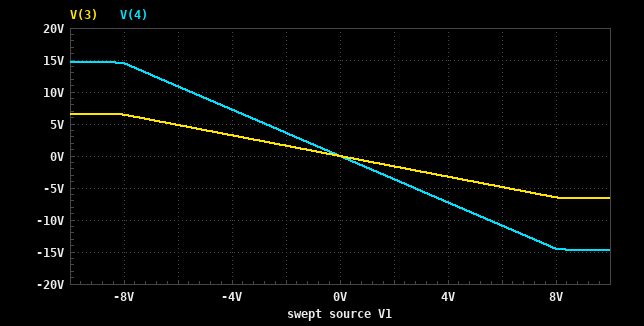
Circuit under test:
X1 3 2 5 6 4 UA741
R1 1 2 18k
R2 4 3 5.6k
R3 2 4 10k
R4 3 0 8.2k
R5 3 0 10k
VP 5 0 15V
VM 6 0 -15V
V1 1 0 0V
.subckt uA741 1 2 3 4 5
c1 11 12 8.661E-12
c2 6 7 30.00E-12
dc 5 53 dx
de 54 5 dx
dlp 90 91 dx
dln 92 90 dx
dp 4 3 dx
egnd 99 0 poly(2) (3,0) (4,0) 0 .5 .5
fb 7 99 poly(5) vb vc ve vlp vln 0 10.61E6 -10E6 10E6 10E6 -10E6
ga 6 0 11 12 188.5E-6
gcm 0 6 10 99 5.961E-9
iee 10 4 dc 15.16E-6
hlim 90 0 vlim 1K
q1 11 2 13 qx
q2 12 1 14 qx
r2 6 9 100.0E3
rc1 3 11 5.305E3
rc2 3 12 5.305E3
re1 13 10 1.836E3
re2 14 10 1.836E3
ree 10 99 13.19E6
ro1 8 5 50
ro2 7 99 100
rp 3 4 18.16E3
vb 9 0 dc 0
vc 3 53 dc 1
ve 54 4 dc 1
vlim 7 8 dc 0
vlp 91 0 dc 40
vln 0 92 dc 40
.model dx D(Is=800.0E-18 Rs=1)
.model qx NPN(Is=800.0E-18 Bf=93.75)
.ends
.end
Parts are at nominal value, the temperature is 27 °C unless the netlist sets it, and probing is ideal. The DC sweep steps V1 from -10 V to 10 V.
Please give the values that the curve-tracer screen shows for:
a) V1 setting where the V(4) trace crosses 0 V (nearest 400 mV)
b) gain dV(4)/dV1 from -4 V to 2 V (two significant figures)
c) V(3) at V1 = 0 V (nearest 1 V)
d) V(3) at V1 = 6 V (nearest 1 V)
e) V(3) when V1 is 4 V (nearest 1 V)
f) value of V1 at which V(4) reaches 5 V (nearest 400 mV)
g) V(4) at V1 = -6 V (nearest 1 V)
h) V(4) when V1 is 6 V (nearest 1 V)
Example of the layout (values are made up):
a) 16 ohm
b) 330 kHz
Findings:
a) 0 V
b) -1.8 V/V
c) 0 V
d) -5 V
e) -3 V
f) -2.8 V
g) 11 V
h) -11 V
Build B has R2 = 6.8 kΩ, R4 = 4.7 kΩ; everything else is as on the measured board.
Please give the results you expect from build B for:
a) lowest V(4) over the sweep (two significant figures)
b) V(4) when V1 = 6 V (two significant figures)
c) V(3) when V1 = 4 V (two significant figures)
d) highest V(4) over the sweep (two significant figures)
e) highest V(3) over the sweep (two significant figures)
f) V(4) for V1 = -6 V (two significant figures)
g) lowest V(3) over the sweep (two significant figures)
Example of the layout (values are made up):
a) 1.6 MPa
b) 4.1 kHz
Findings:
a) -11 V
b) -6.6 V
c) -1.4 V
d) 11 V
e) 3.5 V
f) 6.6 V
g) -3.5 V
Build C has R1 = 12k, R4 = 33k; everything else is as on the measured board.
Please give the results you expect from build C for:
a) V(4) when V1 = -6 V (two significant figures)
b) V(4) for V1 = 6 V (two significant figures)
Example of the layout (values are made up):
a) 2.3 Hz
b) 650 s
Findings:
a) 15 V
b) -15 V
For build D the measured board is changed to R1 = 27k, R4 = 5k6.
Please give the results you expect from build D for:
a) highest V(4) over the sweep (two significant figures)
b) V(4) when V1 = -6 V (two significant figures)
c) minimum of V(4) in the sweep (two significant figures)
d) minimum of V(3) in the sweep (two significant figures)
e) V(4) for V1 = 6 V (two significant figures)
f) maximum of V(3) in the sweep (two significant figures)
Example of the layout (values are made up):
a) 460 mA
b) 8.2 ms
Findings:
a) 8.0 V
b) 4.8 V
c) -8.0 V
d) -3.1 V
e) -4.8 V
f) 3.1 V
